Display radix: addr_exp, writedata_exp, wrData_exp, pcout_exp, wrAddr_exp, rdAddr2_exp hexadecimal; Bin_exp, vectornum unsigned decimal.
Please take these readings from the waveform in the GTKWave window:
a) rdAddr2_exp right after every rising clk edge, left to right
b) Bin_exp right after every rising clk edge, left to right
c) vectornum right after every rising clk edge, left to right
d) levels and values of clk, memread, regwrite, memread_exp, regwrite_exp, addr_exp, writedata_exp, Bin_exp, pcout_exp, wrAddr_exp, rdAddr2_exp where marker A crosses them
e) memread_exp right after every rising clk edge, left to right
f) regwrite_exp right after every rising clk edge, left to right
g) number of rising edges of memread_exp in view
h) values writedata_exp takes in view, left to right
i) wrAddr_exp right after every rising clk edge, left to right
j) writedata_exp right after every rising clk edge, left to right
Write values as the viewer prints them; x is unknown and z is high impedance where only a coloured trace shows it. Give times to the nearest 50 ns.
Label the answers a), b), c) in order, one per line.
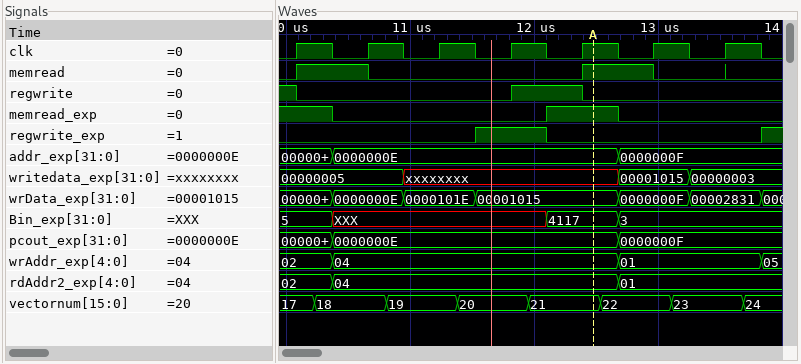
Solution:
a) 02, 04, 04, 04, 04, 01, 01
b) 5, XXX, XXX, XXX, 4117, 3, 3
c) 17, 18, 19, 20, 21, 22, 23
d) clk=1, memread=1, regwrite=0, memread_exp=1, regwrite_exp=0, addr_exp=0000000E, writedata_exp=xxxxxxxx, Bin_exp=4117, pcout_exp=0000000E, wrAddr_exp=04, rdAddr2_exp=04
e) 1 0 0 0 1 0 0
f) 0 0 0 1 0 0 0
g) 1
h) 00000005, xxxxxxxx, 00001015, 00000003
i) 02, 04, 04, 04, 04, 01, 01
j) 00000005, 00000005, xxxxxxxx, xxxxxxxx, xxxxxxxx, 00001015, 00000003
